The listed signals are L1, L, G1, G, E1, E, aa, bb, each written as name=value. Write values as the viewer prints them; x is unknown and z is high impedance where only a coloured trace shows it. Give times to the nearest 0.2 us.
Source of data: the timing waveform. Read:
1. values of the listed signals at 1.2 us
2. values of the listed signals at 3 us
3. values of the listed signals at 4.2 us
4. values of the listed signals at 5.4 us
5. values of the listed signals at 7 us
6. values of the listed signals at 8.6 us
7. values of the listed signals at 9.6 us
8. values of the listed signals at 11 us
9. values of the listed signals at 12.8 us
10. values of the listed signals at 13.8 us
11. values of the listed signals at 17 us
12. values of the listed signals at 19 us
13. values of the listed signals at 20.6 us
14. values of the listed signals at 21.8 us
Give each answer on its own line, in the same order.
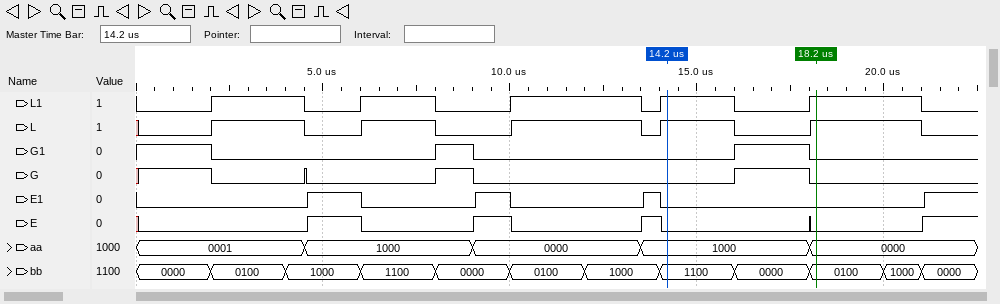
L1=0, L=0, G1=1, G=1, E1=0, E=0, aa=0001, bb=0000
L1=1, L=1, G1=0, G=0, E1=0, E=0, aa=0001, bb=0100
L1=1, L=1, G1=0, G=0, E1=0, E=0, aa=0001, bb=1000
L1=0, L=0, G1=0, G=0, E1=1, E=1, aa=1000, bb=1000
L1=1, L=1, G1=0, G=0, E1=0, E=0, aa=1000, bb=1100
L1=0, L=0, G1=1, G=1, E1=0, E=0, aa=1000, bb=0000
L1=0, L=0, G1=0, G=0, E1=1, E=1, aa=0000, bb=0000
L1=1, L=1, G1=0, G=0, E1=0, E=0, aa=0000, bb=0100
L1=1, L=1, G1=0, G=0, E1=0, E=0, aa=0000, bb=1000
L1=0, L=0, G1=0, G=0, E1=1, E=1, aa=1000, bb=1000
L1=0, L=0, G1=1, G=1, E1=0, E=0, aa=1000, bb=0000
L1=1, L=1, G1=0, G=0, E1=0, E=0, aa=0000, bb=0100
L1=1, L=1, G1=0, G=0, E1=0, E=0, aa=0000, bb=1000
L1=0, L=0, G1=0, G=0, E1=1, E=1, aa=0000, bb=0000
